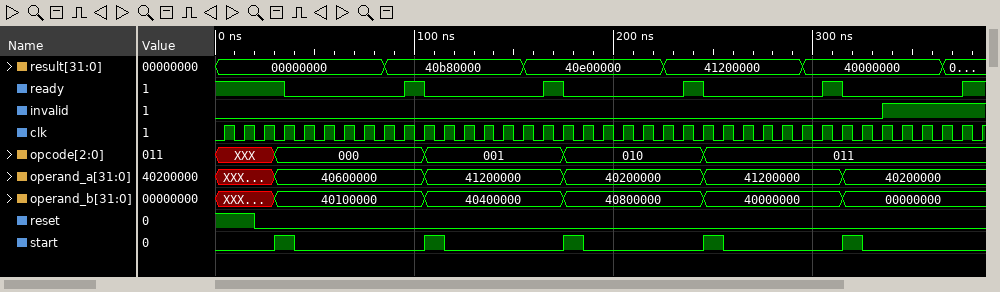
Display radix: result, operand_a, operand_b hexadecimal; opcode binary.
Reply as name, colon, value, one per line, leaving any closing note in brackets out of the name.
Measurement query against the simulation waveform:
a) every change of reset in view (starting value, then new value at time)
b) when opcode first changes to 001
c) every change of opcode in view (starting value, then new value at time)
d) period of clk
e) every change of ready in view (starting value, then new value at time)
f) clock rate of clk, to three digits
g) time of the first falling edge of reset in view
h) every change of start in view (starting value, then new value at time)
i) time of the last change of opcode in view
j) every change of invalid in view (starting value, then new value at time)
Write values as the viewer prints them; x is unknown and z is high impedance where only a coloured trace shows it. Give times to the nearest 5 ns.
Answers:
every change of reset in view: 1, 0 at 20 ns
when opcode first changes to 001: 105 ns
every change of opcode in view: XXX, 000 at 30 ns, 001 at 105 ns, 010 at 175 ns, 011 at 245 ns
period of clk: 10 ns
every change of ready in view: 1, 0 at 35 ns, 1 at 95 ns, 0 at 105 ns, 1 at 165 ns, 0 at 175 ns, 1 at 235 ns, 0 at 245 ns, 1 at 305 ns, 0 at 315 ns, 1 at 375 ns
clock rate of clk, to three digits: 100 MHz
time of the first falling edge of reset in view: 20 ns
every change of start in view: 0, 1 at 30 ns, 0 at 40 ns, 1 at 105 ns, 0 at 115 ns, 1 at 175 ns, 0 at 185 ns, 1 at 245 ns, 0 at 255 ns, 1 at 315 ns, 0 at 325 ns
time of the last change of opcode in view: 245 ns
every change of invalid in view: 0, 1 at 335 ns
